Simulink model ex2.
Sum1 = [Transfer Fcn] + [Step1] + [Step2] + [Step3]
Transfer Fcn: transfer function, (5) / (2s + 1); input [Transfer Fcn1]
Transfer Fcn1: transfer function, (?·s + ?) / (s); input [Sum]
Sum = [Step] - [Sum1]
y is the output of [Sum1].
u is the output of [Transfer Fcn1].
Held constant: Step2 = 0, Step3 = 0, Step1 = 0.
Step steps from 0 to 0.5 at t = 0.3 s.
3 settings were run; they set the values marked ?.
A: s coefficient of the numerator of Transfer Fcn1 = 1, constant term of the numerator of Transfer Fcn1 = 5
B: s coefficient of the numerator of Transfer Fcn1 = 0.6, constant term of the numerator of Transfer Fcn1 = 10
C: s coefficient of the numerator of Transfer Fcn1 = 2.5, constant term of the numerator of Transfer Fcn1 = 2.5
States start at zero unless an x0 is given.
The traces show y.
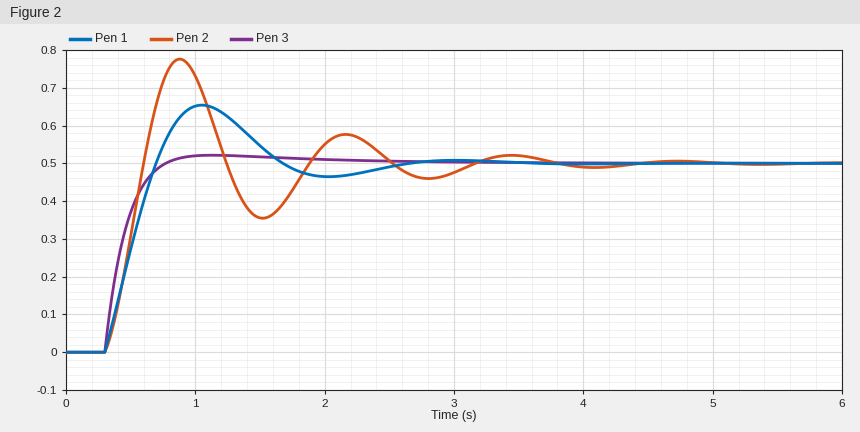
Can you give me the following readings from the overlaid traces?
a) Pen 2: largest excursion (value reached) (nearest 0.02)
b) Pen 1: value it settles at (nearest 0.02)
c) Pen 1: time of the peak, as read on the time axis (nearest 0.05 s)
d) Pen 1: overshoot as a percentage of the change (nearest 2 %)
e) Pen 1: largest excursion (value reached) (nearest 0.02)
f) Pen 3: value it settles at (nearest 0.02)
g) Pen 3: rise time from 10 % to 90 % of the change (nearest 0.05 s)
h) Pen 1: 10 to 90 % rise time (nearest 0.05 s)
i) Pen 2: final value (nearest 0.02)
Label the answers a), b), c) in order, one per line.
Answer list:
a) 0.78
b) 0.50
c) 1.05 s
d) 30 %
e) 0.66
f) 0.50
g) 0.30 s
h) 0.30 s
i) 0.50
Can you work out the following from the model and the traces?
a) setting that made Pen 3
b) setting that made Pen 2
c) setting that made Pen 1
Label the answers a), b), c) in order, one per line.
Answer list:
a) C
b) B
c) A
